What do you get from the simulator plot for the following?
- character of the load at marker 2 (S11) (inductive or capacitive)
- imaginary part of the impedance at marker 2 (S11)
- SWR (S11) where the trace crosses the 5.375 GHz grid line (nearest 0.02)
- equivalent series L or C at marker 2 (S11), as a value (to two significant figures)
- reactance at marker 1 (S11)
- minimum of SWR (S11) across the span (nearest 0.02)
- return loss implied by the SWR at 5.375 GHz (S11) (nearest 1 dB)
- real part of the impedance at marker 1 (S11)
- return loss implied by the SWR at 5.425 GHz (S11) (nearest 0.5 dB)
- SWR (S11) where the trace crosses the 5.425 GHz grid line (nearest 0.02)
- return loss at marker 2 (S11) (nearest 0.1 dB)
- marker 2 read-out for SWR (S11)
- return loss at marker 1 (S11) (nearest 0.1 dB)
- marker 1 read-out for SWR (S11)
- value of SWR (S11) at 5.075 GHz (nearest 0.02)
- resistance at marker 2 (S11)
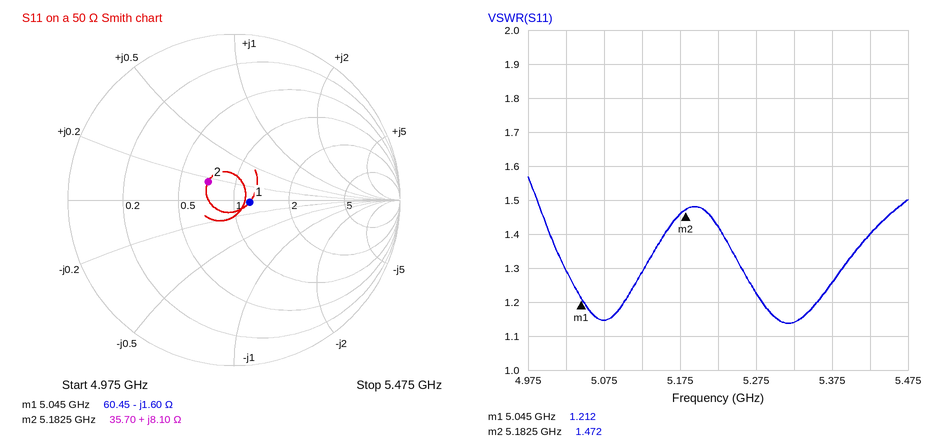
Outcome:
inductive
+8.10 Ω
1.26
250 pH
-1.60 Ω
1.14
19 dB
60.45 Ω
15.5 dB
1.40
14.4 dB
1.472
20.4 dB
1.212
1.14
35.70 Ω
